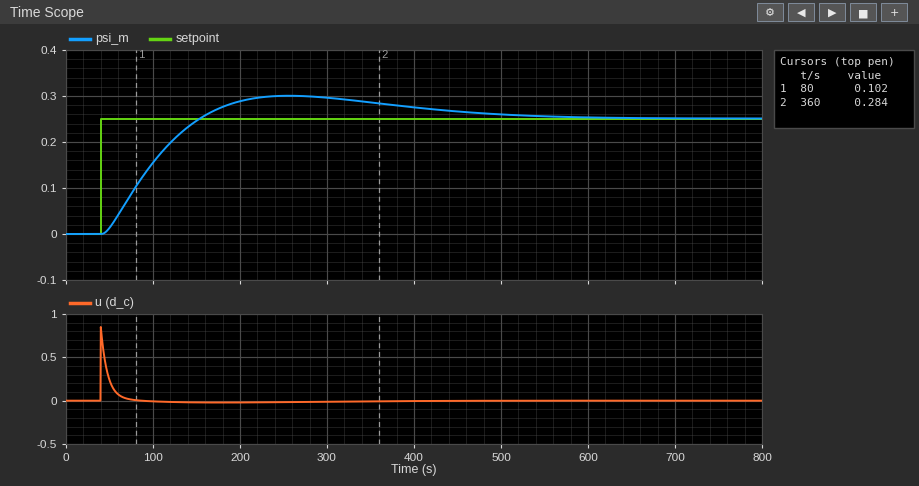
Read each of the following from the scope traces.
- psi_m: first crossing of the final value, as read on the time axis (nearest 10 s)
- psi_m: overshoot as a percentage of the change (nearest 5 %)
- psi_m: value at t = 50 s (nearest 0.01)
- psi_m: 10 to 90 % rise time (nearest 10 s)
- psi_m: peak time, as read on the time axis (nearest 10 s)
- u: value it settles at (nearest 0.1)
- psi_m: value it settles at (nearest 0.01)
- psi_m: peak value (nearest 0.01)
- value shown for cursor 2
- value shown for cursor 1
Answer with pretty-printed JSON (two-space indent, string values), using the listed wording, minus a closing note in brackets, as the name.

{
  "psi_m: first crossing of the final value, as read on the time axis": "150 s",
  "psi_m: overshoot as a percentage of the change": "20 %",
  "psi_m: value at t = 50 s": "0.01",
  "psi_m: 10 to 90 % rise time": "80 s",
  "psi_m: peak time, as read on the time axis": "260 s",
  "u: value it settles at": "0.0",
  "psi_m: value it settles at": "0.25",
  "psi_m: peak value": "0.30",
  "value shown for cursor 2": "0.284",
  "value shown for cursor 1": "0.102"
}
